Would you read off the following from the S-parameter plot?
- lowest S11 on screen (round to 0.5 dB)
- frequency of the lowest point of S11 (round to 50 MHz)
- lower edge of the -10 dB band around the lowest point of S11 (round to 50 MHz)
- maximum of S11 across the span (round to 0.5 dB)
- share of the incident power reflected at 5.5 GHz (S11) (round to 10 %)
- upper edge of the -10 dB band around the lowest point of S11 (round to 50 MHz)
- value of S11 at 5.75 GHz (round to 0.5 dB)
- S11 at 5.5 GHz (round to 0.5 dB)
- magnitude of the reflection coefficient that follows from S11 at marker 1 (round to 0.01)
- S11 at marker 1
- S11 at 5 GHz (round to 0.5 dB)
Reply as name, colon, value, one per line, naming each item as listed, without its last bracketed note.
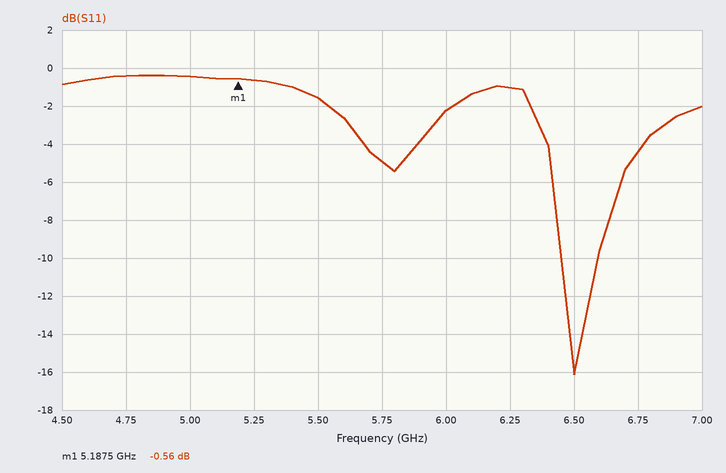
lowest S11 on screen: -16.0 dB
frequency of the lowest point of S11: 6.50 GHz
lower edge of the -10 dB band around the lowest point of S11: 6.45 GHz
maximum of S11 across the span: -0.5 dB
share of the incident power reflected at 5.5 GHz (S11): 70 %
upper edge of the -10 dB band around the lowest point of S11: 6.60 GHz
value of S11 at 5.75 GHz: -5.0 dB
S11 at 5.5 GHz: -1.5 dB
magnitude of the reflection coefficient that follows from S11 at marker 1: 0.94
S11 at marker 1: -0.56 dB
S11 at 5 GHz: -0.5 dB
